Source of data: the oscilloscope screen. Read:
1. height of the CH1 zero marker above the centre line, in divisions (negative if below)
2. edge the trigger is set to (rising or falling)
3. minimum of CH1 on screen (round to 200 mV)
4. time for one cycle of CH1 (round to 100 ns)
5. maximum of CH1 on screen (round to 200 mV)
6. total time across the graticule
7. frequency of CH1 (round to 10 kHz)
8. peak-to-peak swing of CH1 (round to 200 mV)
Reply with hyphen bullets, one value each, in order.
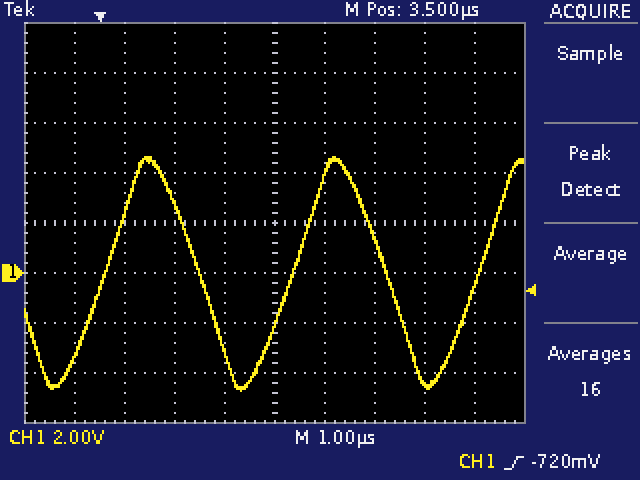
- -1.0 div
- rising
- -4.8 V
- 3.7 µs
- 4.6 V
- 10 µs
- 270 kHz
- 9.4 V
